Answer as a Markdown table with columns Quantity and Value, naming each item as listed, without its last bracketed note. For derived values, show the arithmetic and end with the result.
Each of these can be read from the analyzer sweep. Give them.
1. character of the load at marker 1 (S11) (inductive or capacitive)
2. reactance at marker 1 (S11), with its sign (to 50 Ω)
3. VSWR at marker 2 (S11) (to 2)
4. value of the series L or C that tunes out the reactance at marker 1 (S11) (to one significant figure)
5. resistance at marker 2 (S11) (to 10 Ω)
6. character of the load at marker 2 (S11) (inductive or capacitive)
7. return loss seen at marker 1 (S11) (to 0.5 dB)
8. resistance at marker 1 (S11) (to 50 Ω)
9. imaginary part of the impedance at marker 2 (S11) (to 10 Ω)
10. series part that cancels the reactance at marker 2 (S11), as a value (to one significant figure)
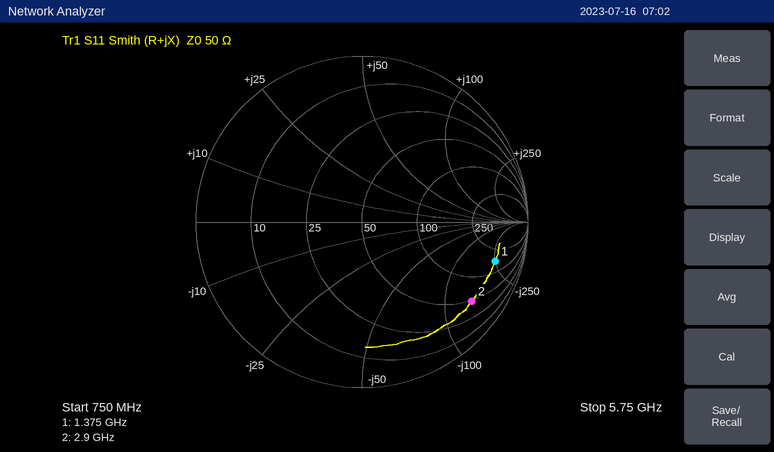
| Quantity | Value |
|---|---|
| character of the load at marker 1 (S11) | capacitive |
| reactance at marker 1 (S11), with its sign | -250 Ω |
| VSWR at marker 2 (S11) | 10 |
| value of the series L or C that tunes out the reactance at marker 1 (S11) | L = 250 Ω/(2π × 1.375 GHz) ≈ 28.9 nH, so 30 nH to one significant figure |
| resistance at marker 2 (S11) | 50 Ω |
| character of the load at marker 2 (S11) | capacitive |
| return loss seen at marker 1 (S11) | 1.5 dB |
| resistance at marker 1 (S11) | 150 Ω |
| imaginary part of the impedance at marker 2 (S11) | -140 Ω |
| series part that cancels the reactance at marker 2 (S11), as a value | L = 140 Ω/(2π × 2.9 GHz) ≈ 8 nH |
